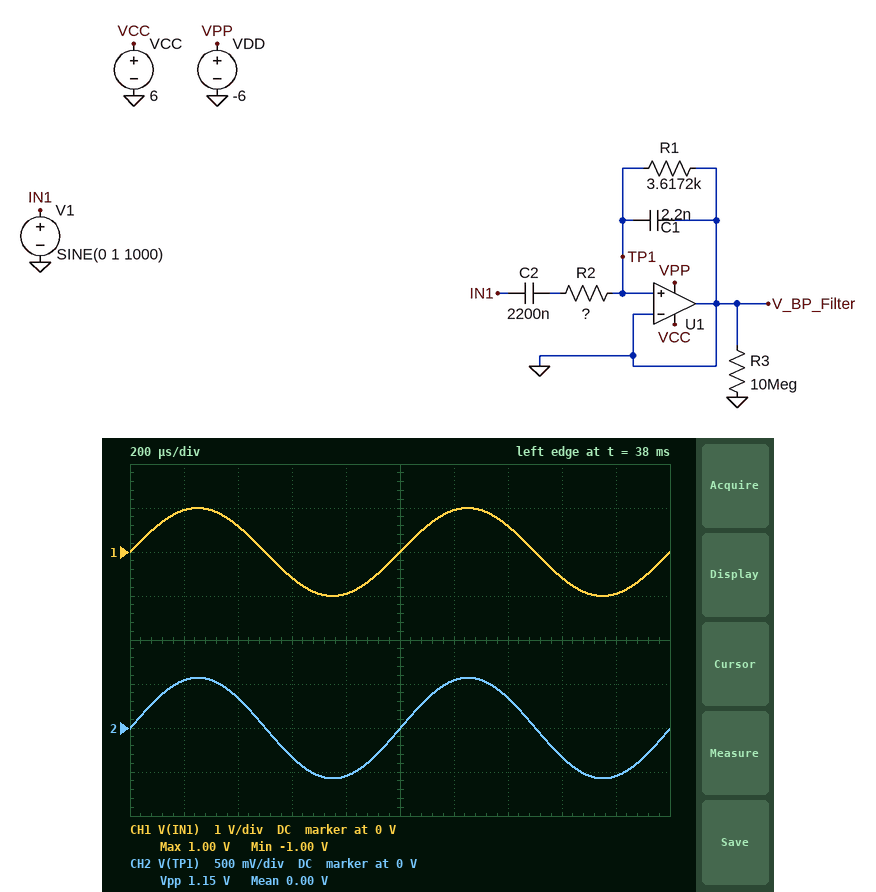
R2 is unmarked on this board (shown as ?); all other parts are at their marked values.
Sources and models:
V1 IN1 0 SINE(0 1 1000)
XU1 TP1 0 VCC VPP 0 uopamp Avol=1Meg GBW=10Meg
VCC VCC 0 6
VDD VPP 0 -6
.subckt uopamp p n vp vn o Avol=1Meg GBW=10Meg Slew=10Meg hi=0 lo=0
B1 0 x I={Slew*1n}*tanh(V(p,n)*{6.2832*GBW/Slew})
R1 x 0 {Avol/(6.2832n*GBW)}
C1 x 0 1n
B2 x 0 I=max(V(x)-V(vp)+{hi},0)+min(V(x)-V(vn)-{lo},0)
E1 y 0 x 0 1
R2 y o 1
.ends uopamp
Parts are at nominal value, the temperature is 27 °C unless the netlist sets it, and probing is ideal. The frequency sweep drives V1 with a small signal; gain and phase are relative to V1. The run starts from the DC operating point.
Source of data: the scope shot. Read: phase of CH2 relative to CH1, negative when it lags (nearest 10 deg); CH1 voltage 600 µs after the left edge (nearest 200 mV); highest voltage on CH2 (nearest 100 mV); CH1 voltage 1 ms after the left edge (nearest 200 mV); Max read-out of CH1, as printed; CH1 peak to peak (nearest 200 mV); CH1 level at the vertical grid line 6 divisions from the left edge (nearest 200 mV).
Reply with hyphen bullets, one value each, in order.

- 0 deg
- -600 mV
- 600 mV
- 0 V
- 1.00 V
- 2.0 V
- 1.0 V
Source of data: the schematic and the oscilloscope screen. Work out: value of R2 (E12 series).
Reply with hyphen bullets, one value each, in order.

- 2.7 kΩ
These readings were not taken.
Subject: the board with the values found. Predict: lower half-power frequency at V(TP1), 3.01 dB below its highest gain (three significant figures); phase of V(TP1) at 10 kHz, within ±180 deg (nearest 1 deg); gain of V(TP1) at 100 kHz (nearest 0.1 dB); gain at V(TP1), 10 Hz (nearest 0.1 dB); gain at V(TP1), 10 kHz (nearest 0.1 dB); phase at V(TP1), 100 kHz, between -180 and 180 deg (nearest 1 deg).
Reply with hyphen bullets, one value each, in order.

- 11.4 Hz
- -12 deg
- -12.3 dB
- -8.5 dB
- -5.0 dB
- -65 deg
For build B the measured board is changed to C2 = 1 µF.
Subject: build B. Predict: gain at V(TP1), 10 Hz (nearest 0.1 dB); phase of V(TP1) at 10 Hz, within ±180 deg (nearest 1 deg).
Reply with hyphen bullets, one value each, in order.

- -13.5 dB
- 68 deg
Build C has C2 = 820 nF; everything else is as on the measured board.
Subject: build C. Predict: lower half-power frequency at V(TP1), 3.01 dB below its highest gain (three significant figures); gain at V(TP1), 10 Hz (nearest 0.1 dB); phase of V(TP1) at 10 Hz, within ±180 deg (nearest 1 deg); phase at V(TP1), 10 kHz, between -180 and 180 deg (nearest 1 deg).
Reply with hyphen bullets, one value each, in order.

- 30.7 Hz
- -15.0 dB
- 72 deg
- -12 deg
